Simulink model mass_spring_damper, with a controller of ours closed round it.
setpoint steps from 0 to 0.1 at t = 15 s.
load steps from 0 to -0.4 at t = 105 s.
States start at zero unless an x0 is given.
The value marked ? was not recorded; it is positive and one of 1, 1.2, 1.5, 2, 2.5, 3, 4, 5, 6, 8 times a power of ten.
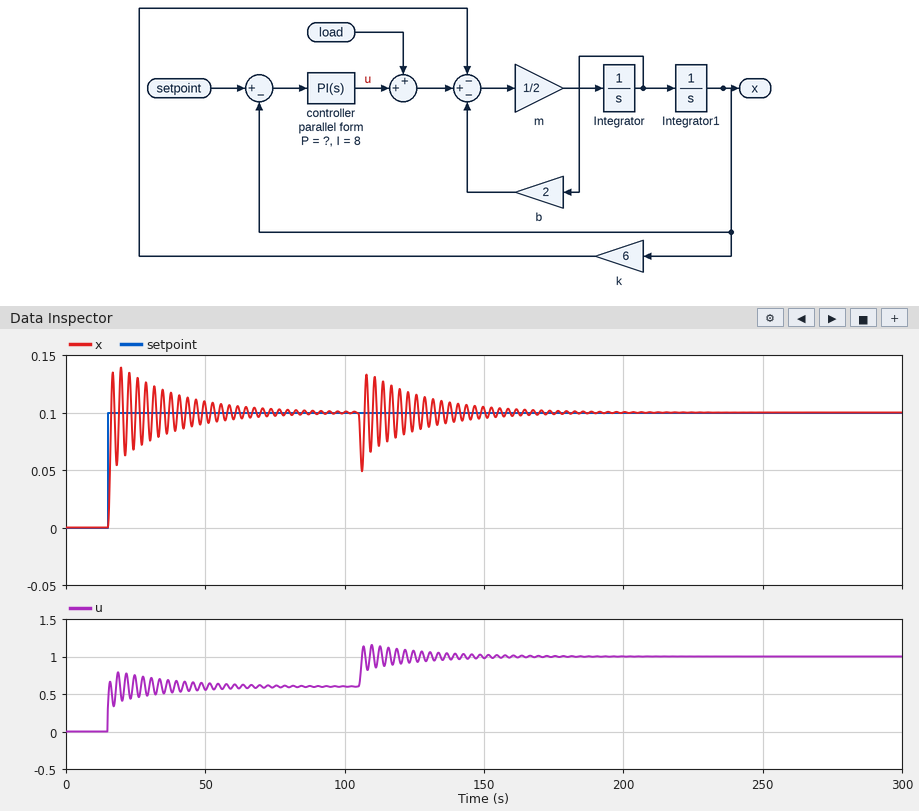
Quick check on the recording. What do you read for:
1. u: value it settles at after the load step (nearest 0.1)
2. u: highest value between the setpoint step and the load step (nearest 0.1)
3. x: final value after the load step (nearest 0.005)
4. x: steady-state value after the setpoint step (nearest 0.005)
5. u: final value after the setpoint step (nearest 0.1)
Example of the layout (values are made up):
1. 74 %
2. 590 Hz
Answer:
1. 1.0
2. 0.8
3. 0.100
4. 0.100
5. 0.6
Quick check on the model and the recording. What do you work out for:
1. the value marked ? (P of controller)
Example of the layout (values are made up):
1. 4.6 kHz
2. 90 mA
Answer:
1. 3
